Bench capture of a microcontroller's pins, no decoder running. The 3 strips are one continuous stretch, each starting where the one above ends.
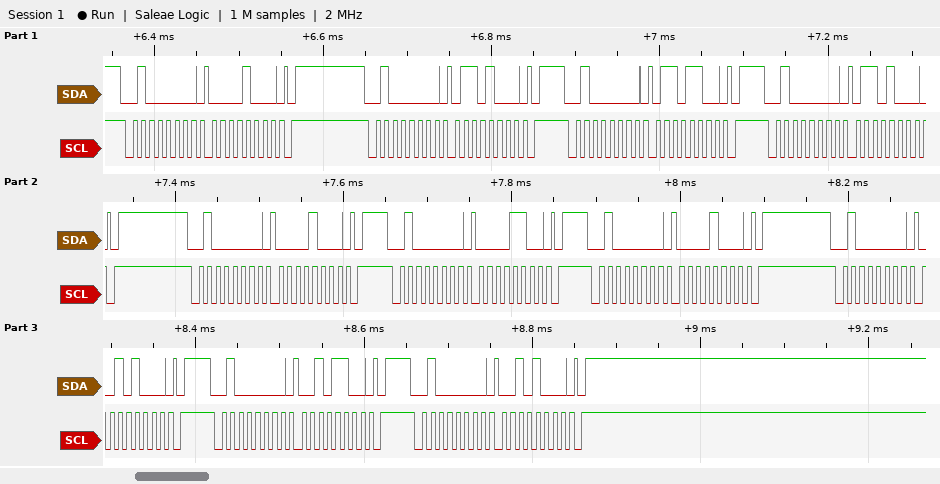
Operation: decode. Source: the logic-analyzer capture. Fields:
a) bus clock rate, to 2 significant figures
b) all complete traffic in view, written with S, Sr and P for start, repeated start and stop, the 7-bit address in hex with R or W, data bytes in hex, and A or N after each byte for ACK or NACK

100 kHz
S 20W A 08 A P S 20W A 68 A P S 20W A 6C A P S 20W A 68 A P S 20W A 08 A P S 20W A 0C A P S 20W A 08 A P S 20W A 28 A P S 20W A 2C A P S 20W A 28 A P
